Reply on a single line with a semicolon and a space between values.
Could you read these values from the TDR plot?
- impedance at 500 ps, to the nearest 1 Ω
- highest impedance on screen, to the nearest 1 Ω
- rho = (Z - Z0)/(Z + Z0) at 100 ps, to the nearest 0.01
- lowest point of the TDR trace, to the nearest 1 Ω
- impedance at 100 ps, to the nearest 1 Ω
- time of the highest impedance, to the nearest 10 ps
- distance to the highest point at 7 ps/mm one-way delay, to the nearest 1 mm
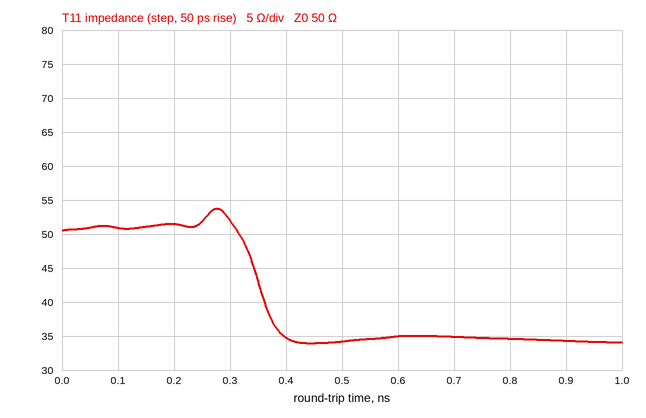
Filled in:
34 Ω; 54 Ω; +0.01; 34 Ω; 51 Ω; 280 ps; 20 mm
